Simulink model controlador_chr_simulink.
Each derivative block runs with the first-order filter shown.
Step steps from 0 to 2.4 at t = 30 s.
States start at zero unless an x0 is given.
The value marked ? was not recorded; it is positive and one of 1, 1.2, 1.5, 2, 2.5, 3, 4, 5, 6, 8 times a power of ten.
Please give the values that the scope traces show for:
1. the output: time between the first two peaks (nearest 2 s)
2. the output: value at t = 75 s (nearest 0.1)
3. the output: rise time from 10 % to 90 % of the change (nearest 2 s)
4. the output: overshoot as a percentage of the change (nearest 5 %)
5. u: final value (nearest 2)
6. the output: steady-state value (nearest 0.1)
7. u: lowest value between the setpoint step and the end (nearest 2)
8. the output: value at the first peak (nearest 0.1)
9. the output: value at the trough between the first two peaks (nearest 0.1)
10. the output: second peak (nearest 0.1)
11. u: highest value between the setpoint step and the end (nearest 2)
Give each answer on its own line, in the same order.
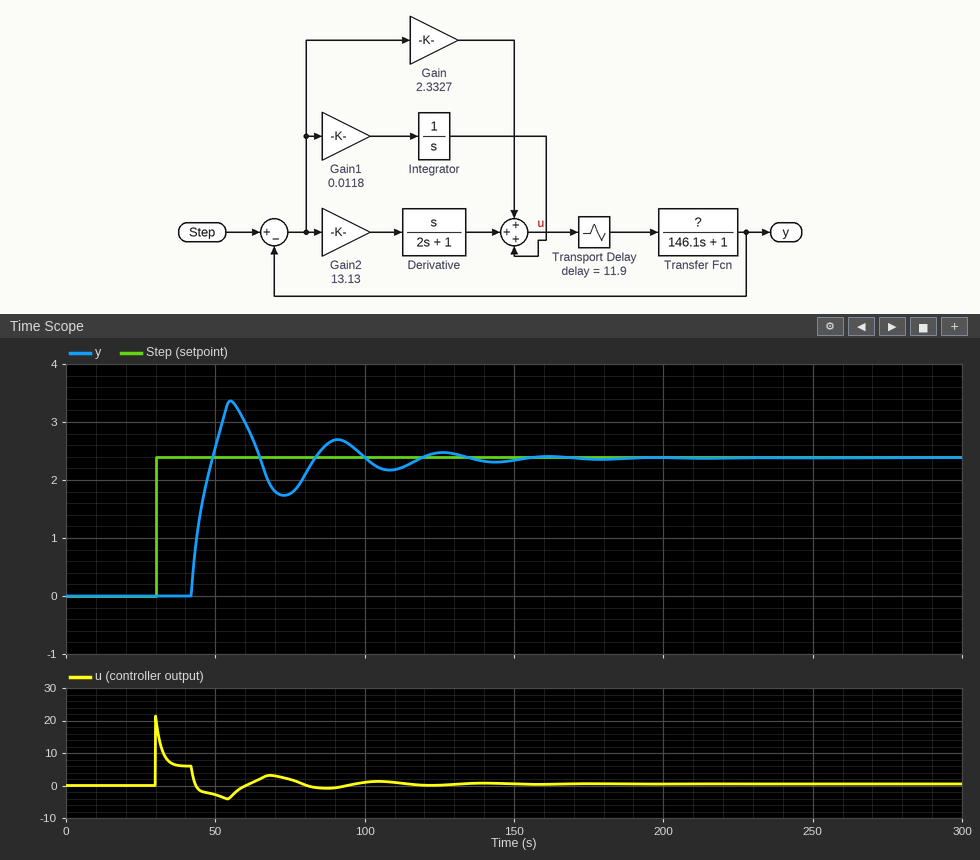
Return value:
36 s
1.8
6 s
40 %
0
2.4
-4
3.4
1.7
2.7
22
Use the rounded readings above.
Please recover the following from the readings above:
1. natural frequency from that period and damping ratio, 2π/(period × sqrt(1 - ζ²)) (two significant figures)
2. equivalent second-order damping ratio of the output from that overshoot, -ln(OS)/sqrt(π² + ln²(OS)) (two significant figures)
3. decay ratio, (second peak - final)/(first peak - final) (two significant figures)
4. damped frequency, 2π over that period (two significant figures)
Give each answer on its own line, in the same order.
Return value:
0.18 rad/s
0.28
0.30
0.17 rad/s
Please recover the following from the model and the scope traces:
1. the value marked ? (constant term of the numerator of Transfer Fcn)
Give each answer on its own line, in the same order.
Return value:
5
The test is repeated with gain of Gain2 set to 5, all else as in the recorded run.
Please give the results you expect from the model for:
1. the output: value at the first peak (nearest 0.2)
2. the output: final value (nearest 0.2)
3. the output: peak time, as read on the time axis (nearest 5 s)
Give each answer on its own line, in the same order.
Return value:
3.2
2.4
60 s
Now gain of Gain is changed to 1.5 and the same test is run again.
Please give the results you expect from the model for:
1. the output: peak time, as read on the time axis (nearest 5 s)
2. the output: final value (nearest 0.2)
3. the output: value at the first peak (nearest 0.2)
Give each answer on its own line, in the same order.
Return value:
55 s
2.4
2.6
